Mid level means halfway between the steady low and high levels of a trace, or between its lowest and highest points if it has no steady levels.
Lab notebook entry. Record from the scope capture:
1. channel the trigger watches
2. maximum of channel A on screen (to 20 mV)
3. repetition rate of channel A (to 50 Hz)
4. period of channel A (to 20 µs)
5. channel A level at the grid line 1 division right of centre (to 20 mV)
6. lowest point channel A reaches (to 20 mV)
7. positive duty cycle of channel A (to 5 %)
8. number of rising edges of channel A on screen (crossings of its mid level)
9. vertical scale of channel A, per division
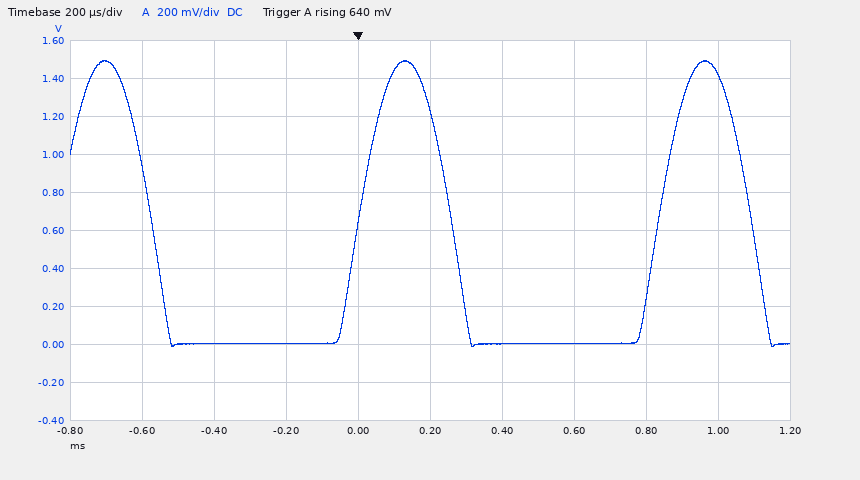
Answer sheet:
channel A
1.50 V
1.20 kHz
840 µs
0 mV
-20 mV
30 %
2
200 mV
